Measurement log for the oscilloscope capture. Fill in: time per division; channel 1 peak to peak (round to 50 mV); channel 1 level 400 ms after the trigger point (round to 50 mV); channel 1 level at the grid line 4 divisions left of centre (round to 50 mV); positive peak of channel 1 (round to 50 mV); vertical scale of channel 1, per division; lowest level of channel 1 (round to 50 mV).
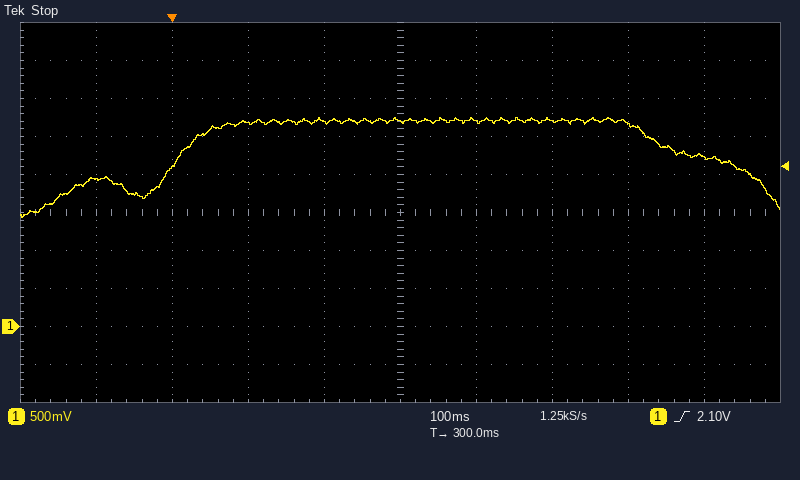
100 ms
1.30 V
2.70 V
1.95 V
2.75 V
500 mV
1.45 V
